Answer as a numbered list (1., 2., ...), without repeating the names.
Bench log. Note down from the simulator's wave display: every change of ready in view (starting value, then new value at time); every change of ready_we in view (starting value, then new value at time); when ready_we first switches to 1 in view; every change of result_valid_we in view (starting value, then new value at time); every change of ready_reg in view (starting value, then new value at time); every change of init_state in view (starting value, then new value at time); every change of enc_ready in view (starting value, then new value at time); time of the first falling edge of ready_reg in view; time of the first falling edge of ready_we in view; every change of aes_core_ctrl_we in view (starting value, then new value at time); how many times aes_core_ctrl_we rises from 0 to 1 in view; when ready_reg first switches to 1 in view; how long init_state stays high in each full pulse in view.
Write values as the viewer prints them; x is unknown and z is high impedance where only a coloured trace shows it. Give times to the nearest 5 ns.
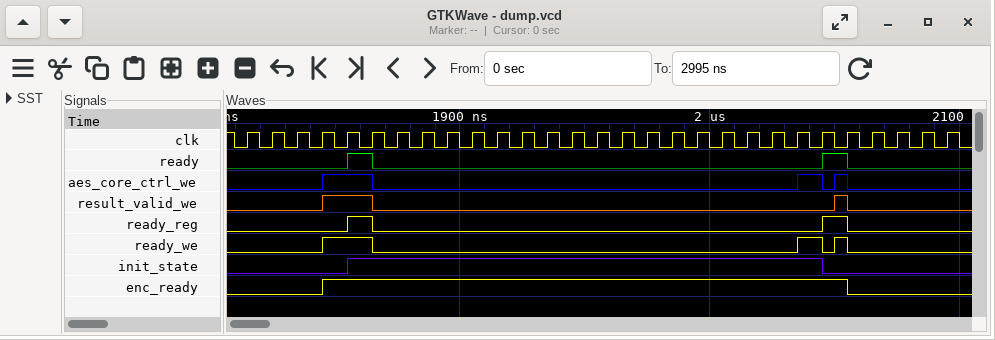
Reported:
1. 0, 1 at 1855 ns, 0 at 1865 ns, 1 at 2045 ns, 0 at 2055 ns
2. 0, 1 at 1845 ns, 0 at 1865 ns, 1 at 2035 ns, 0 at 2045 ns, 1 at 2050 ns, 0 at 2055 ns
3. 1845 ns
4. 0, 1 at 1845 ns, 0 at 1865 ns, 1 at 2050 ns, 0 at 2055 ns
5. 0, 1 at 1855 ns, 0 at 1865 ns, 1 at 2045 ns, 0 at 2055 ns
6. 0, 1 at 1855 ns, 0 at 2045 ns
7. 0, 1 at 1845 ns, 0 at 2055 ns
8. 1865 ns
9. 1865 ns
10. 0, 1 at 1845 ns, 0 at 1865 ns, 1 at 2035 ns, 0 at 2045 ns, 1 at 2050 ns, 0 at 2055 ns
11. 3
12. 1855 ns
13. 190 ns
